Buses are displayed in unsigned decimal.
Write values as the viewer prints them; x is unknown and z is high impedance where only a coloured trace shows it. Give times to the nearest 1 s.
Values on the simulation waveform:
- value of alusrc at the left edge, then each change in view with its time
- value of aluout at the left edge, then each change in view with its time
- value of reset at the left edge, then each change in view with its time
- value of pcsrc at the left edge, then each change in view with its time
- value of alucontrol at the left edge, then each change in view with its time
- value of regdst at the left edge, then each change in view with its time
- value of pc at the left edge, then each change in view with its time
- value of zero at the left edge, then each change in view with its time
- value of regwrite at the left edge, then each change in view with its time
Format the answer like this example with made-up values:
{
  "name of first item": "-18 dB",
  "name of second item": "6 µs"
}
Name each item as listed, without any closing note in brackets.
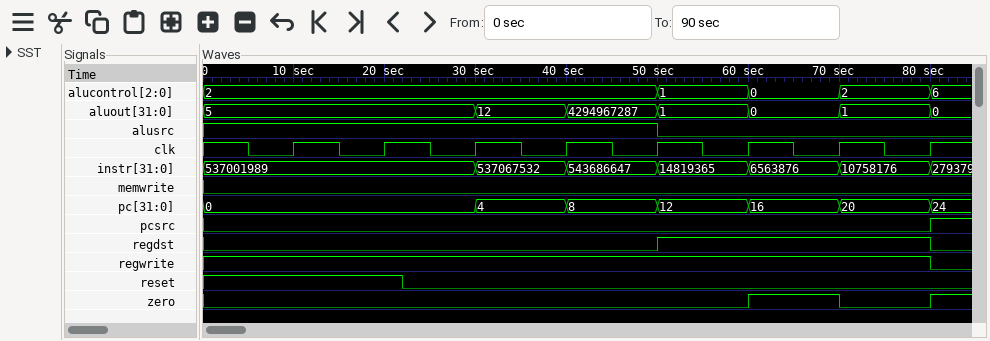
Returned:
{
  "value of alusrc at the left edge, then each change in view with its time": "1, 0 at 50 s",
  "value of aluout at the left edge, then each change in view with its time": "5, 12 at 30 s, 4294967287 at 40 s, 1 at 50 s, 0 at 60 s, 1 at 70 s, 0 at 80 s",
  "value of reset at the left edge, then each change in view with its time": "1, 0 at 22 s",
  "value of pcsrc at the left edge, then each change in view with its time": "0, 1 at 80 s",
  "value of alucontrol at the left edge, then each change in view with its time": "2, 1 at 50 s, 0 at 60 s, 2 at 70 s, 6 at 80 s",
  "value of regdst at the left edge, then each change in view with its time": "0, 1 at 50 s, 0 at 80 s",
  "value of pc at the left edge, then each change in view with its time": "0, 4 at 30 s, 8 at 40 s, 12 at 50 s, 16 at 60 s, 20 at 70 s, 24 at 80 s",
  "value of zero at the left edge, then each change in view with its time": "0, 1 at 60 s, 0 at 70 s, 1 at 80 s",
  "value of regwrite at the left edge, then each change in view with its time": "1, 0 at 80 s"
}
